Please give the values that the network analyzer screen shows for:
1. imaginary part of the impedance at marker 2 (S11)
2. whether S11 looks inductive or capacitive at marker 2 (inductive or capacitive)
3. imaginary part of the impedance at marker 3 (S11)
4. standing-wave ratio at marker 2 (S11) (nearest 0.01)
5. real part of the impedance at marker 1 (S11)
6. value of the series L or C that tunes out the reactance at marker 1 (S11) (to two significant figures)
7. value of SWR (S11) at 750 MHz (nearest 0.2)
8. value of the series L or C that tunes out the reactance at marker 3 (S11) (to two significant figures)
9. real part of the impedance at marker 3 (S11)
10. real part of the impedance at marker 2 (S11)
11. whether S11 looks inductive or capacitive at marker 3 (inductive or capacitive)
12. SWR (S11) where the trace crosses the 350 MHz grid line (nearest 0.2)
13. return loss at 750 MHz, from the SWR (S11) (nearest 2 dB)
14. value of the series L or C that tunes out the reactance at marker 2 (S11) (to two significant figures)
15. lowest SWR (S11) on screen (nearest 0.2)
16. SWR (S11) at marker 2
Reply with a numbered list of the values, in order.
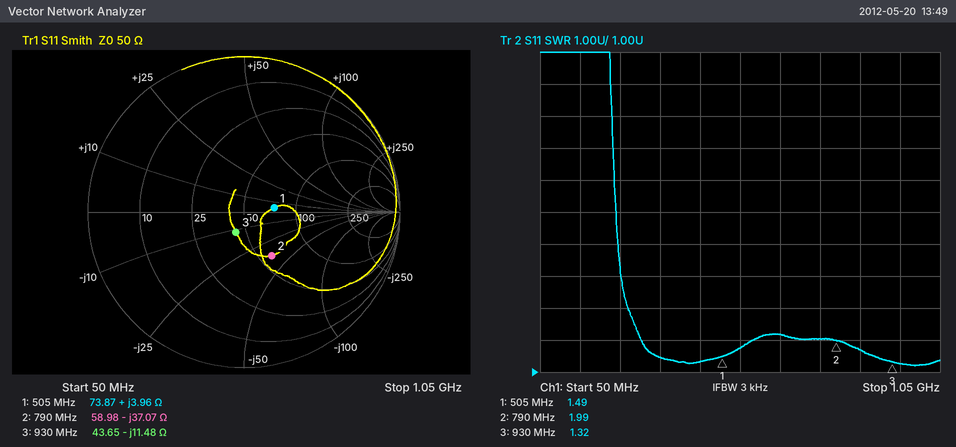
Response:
1. -37.07 Ω
2. capacitive
3. -11.48 Ω
4. 1.99
5. 73.87 Ω
6. 80 pF
7. 2.0
8. 2.0 nH
9. 43.65 Ω
10. 58.98 Ω
11. capacitive
12. 1.4
13. 10 dB
14. 7.5 nH
15. 1.2
16. 1.99
